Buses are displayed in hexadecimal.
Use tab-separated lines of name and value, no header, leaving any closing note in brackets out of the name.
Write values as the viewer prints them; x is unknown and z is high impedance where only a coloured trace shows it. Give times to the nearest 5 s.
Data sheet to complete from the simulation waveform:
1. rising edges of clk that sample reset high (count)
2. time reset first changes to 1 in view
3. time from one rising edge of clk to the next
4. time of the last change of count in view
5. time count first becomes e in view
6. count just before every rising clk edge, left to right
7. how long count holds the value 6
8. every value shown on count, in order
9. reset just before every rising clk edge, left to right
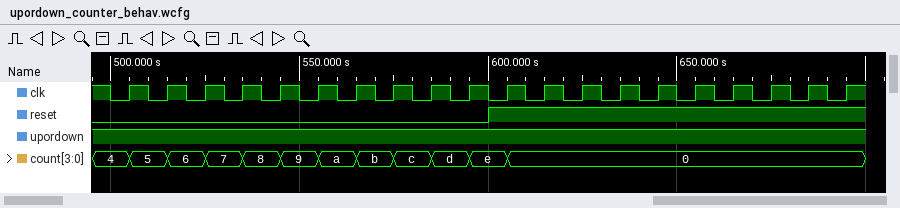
rising edges of clk that sample reset high	10
time reset first changes to 1 in view	600 s
time from one rising edge of clk to the next	10 s
time of the last change of count in view	605 s
time count first becomes e in view	595 s
count just before every rising clk edge, left to right	4, 5, 6, 7, 8, 9, a, b, c, d, e, 0, 0, 0, 0, 0, 0, 0, 0, 0
how long count holds the value 6	10 s
every value shown on count, in order	4, 5, 6, 7, 8, 9, a, b, c, d, e, 0
reset just before every rising clk edge, left to right	0 0 0 0 0 0 0 0 0 0 1 1 1 1 1 1 1 1 1 1
